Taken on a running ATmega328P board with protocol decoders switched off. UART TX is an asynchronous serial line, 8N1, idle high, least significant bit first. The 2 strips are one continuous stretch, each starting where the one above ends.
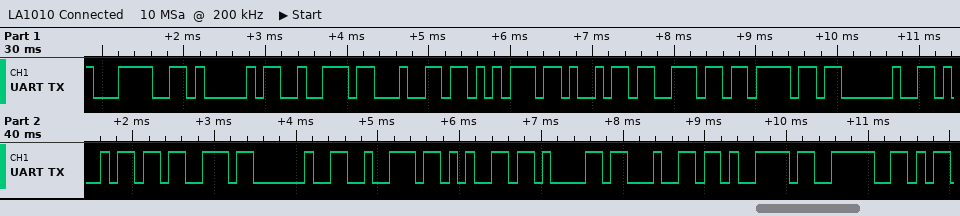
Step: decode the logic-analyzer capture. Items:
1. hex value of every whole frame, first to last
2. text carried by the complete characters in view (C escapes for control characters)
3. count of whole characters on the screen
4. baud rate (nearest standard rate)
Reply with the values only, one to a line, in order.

0x3C 0x41 0x72 0x64 0x75 0x69 0x6E 0x6F 0x20 0x69 0x73 0x20 0x72 0x65 0x61 0x64 0x79 0x3E
"<Arduino is ready>"
18
9600 baud
